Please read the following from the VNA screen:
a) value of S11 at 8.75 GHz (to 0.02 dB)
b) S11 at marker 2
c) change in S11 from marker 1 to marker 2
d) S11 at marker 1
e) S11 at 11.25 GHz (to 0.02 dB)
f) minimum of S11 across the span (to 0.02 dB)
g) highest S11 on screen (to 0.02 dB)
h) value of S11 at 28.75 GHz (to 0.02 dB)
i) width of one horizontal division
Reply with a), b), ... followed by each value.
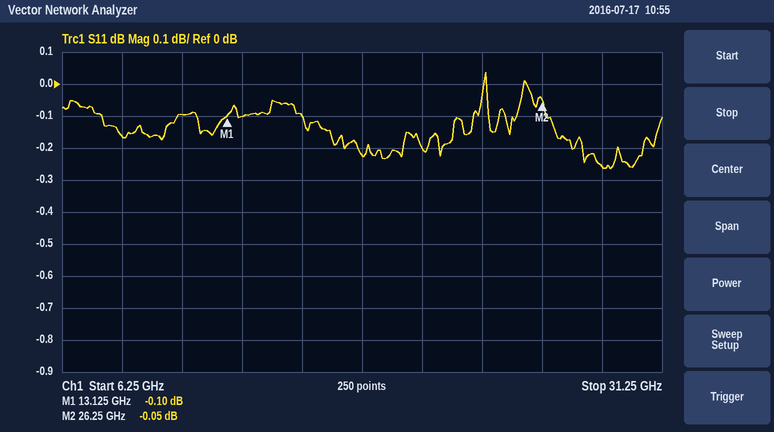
a) -0.16 dB
b) -0.05 dB
c) 0.05 dB
d) -0.10 dB
e) -0.10 dB
f) -0.26 dB
g) 0.04 dB
h) -0.26 dB
i) 2.5 GHz
